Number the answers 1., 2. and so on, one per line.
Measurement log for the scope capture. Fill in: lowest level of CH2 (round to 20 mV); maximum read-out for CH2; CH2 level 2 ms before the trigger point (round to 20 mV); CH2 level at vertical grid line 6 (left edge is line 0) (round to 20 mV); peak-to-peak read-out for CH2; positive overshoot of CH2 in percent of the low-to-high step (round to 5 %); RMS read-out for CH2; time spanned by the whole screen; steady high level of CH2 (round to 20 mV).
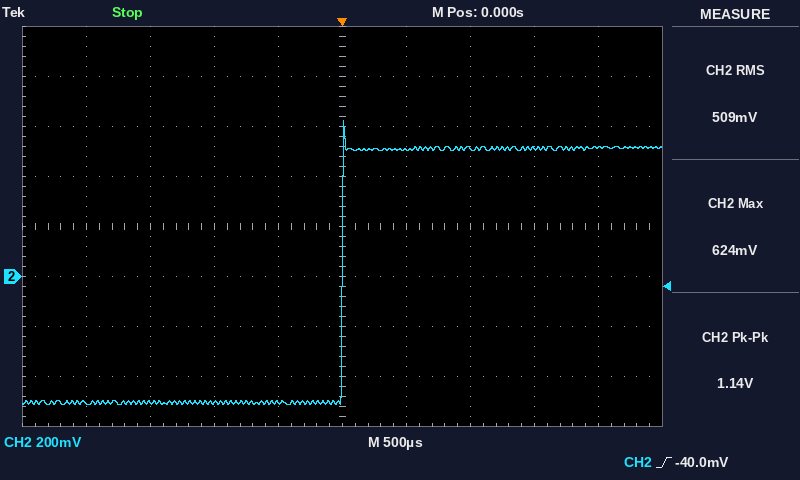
1. -520 mV
2. 624 mV
3. -500 mV
4. 500 mV
5. 1.14 V
6. 10 %
7. 509 mV
8. 5 ms
9. 520 mV
